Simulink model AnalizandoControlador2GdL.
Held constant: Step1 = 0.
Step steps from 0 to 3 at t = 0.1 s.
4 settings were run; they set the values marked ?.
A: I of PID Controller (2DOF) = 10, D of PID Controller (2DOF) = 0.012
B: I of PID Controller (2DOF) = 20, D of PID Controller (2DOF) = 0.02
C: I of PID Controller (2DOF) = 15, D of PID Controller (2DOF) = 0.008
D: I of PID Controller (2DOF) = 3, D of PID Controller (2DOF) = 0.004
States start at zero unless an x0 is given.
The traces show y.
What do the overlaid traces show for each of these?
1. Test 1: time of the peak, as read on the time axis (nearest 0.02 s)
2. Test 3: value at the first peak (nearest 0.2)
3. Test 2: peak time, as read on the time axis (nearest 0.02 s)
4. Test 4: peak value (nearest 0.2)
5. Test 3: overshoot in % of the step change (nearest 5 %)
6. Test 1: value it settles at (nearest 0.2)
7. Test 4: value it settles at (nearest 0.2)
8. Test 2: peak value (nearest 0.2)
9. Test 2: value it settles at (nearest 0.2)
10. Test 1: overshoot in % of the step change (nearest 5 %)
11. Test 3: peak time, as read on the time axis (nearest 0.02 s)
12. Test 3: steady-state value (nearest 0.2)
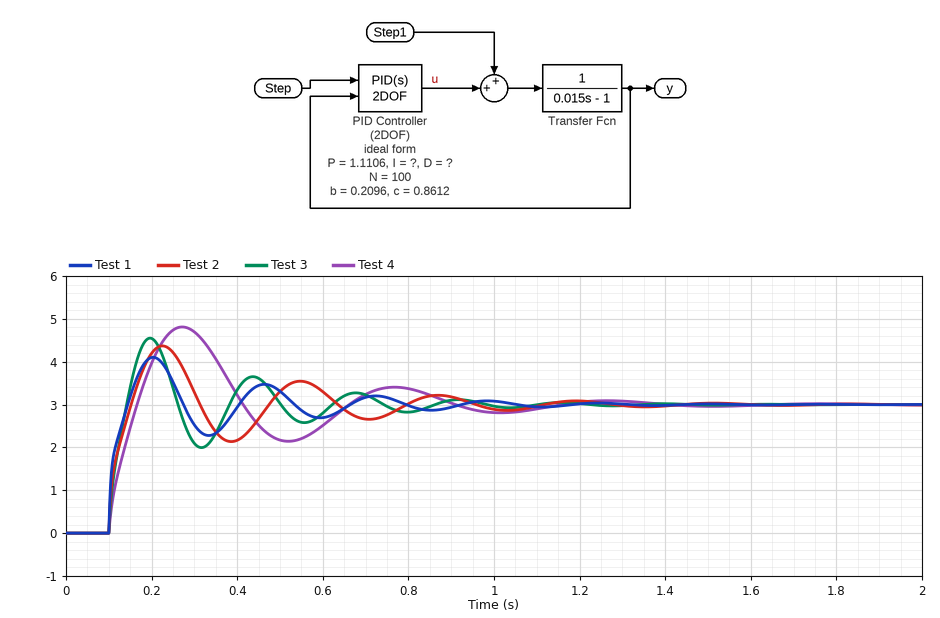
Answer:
0.20 s
4.6
0.22 s
4.8
50 %
3.0
3.0
4.4
3.0
35 %
0.20 s
3.0
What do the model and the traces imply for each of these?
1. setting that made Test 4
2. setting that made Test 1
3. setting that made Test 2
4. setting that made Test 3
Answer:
D
B
A
C
